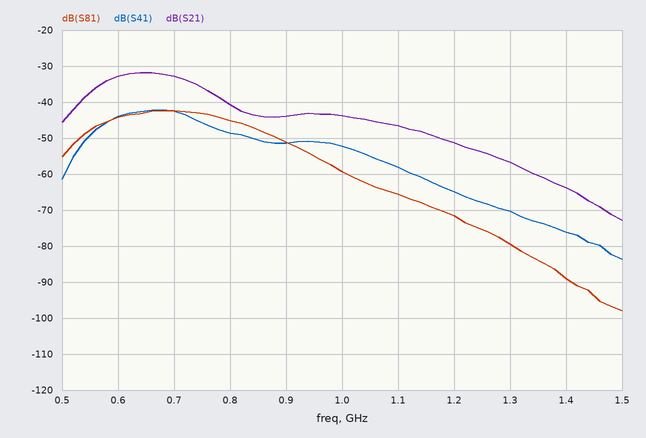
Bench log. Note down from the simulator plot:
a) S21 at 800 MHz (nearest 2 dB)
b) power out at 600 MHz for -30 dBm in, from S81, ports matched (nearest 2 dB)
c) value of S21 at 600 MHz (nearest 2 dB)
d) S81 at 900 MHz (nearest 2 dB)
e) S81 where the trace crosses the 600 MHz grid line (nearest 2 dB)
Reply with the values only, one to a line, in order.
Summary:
-40 dB
-74 dBm
-32 dB
-52 dB
-44 dB
